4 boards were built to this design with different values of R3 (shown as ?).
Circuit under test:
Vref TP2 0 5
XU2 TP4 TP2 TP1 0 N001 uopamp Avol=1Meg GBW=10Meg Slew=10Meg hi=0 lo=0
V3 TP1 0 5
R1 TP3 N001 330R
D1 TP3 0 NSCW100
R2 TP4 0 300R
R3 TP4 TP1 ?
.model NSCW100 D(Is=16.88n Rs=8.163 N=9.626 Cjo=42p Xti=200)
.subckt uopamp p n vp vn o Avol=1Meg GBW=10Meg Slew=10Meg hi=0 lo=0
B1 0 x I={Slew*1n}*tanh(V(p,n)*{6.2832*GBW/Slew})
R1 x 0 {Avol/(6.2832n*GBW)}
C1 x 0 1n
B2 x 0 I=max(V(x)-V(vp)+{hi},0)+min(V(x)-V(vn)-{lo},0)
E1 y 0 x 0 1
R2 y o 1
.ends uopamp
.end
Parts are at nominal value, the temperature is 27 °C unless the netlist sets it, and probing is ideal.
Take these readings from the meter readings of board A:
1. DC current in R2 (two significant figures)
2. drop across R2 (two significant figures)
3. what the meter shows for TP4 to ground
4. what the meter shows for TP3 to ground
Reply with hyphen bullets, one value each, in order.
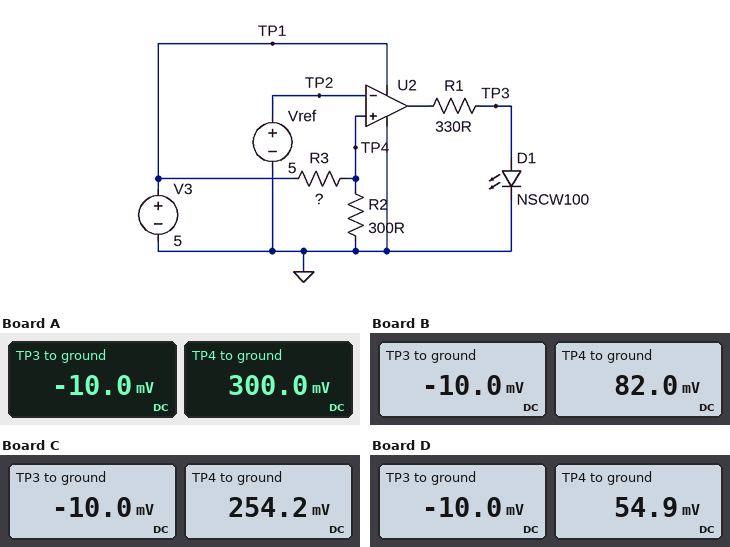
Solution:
- 1.0 mA
- 300 mV
- 300.0 mV
- -10.0 mV
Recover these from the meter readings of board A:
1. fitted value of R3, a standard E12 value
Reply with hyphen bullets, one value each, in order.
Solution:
- 4.7 kΩ
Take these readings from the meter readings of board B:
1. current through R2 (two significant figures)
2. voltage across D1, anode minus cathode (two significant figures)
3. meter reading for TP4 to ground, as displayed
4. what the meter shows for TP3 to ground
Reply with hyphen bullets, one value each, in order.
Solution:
- 270 µA
- -10 mV
- 82.0 mV
- -10.0 mV
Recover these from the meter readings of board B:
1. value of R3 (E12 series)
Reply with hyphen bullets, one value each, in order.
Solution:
- 18 kΩ
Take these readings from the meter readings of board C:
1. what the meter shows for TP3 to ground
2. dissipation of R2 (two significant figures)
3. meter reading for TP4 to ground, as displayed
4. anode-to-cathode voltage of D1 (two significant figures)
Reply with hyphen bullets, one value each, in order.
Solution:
- -10.0 mV
- 220 µW
- 254.2 mV
- -10 mV
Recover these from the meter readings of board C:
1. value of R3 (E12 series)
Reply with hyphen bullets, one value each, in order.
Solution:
- 5.6 kΩ
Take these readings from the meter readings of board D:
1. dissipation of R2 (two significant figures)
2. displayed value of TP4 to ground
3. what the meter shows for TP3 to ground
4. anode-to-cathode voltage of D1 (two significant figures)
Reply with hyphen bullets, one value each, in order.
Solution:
- 10 µW
- 54.9 mV
- -10.0 mV
- -10 mV
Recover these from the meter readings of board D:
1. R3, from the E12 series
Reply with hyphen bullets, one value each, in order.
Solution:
- 27 kΩ
